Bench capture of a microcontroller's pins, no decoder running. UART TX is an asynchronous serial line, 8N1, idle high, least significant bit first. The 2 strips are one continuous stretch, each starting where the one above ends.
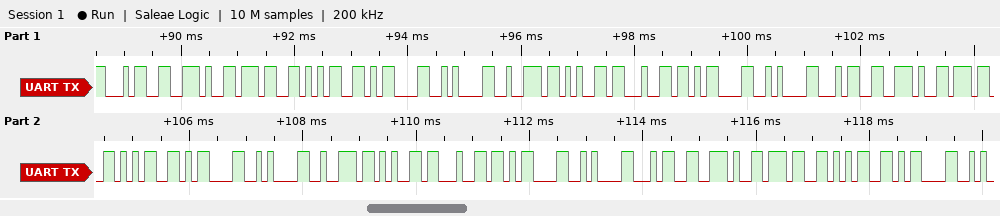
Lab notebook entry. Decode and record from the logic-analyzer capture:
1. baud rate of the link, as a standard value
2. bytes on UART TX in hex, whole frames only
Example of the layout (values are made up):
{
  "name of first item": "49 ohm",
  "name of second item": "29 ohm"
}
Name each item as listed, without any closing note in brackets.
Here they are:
{
  "baud rate of the link, as a standard value": "9600 baud",
  "bytes on UART TX in hex, whole frames only": "0x34 0x2E 0x37 0x35 0x0D 0x0A 0x72 0x65 0x64 0x0D 0x0A 0x34 0x2E 0x37 0x35 0x0D 0x0A 0x72 0x65 0x64 0x0D 0x0A 0x34 0x2E 0x37 0x35 0x0D"
}
